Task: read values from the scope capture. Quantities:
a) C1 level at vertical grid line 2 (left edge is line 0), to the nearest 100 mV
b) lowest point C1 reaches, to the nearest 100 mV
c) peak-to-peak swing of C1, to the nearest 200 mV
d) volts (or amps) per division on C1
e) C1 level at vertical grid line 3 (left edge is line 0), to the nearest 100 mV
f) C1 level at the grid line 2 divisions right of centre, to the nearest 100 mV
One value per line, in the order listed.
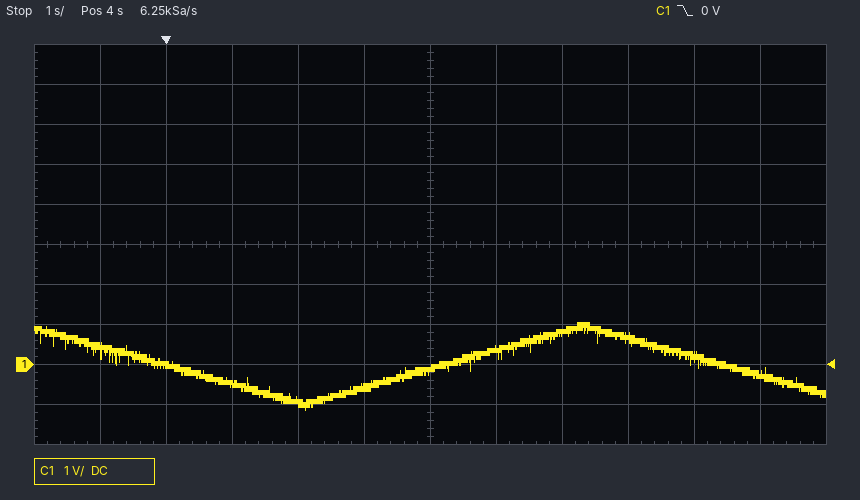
0.0 V
-1.1 V
2.2 V
1 V
-500 mV
800 mV
